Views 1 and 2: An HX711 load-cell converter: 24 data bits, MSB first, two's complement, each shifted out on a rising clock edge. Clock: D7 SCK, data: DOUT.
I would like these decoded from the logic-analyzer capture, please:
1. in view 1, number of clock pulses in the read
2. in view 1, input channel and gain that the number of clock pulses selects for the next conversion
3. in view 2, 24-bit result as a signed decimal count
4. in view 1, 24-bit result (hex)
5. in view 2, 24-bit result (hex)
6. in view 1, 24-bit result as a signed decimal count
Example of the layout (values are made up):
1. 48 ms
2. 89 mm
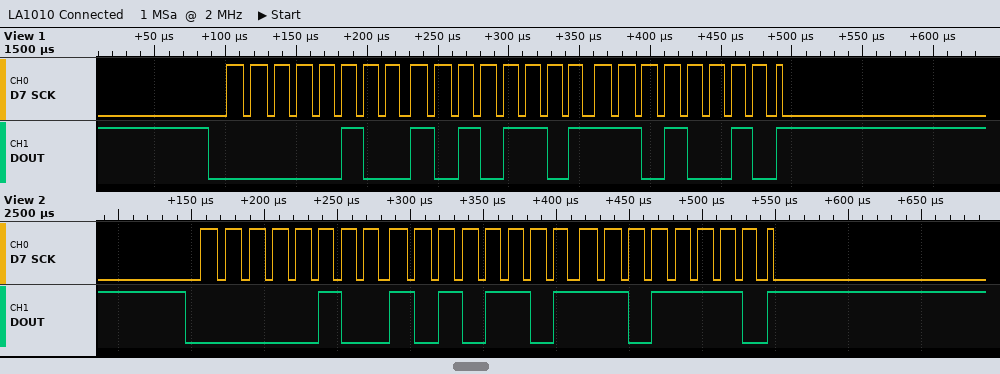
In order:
1. 25
2. channel A, gain 128
3. 306654
4. 0x04ADD2
5. 0x04ADDE
6. 306642
